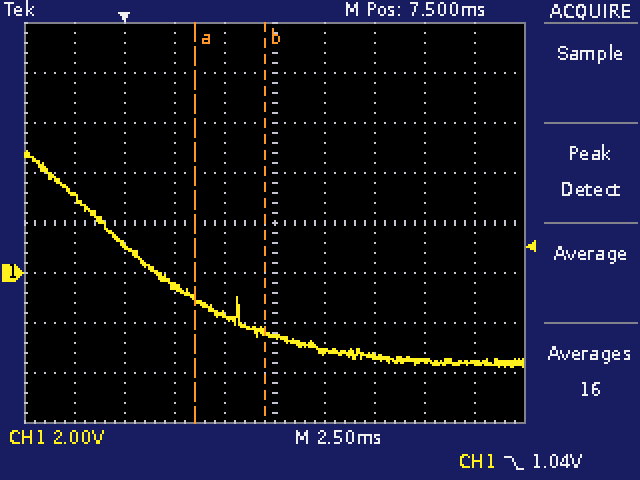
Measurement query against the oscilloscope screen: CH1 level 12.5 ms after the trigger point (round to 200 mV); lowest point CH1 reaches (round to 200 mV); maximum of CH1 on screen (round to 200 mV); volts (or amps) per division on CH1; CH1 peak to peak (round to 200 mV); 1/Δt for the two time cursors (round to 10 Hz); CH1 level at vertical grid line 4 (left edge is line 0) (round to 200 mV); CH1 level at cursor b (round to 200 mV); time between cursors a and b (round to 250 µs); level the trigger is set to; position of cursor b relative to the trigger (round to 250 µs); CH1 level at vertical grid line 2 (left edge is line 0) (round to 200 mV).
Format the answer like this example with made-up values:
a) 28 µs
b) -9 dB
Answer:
a) -3.4 V
b) -3.8 V
c) 4.8 V
d) 2 V
e) 8.6 V
f) 290 Hz
g) -1.6 V
h) -2.4 V
i) 3.50 ms
j) 1.04 V
k) +7.00 ms
l) 1.2 V
